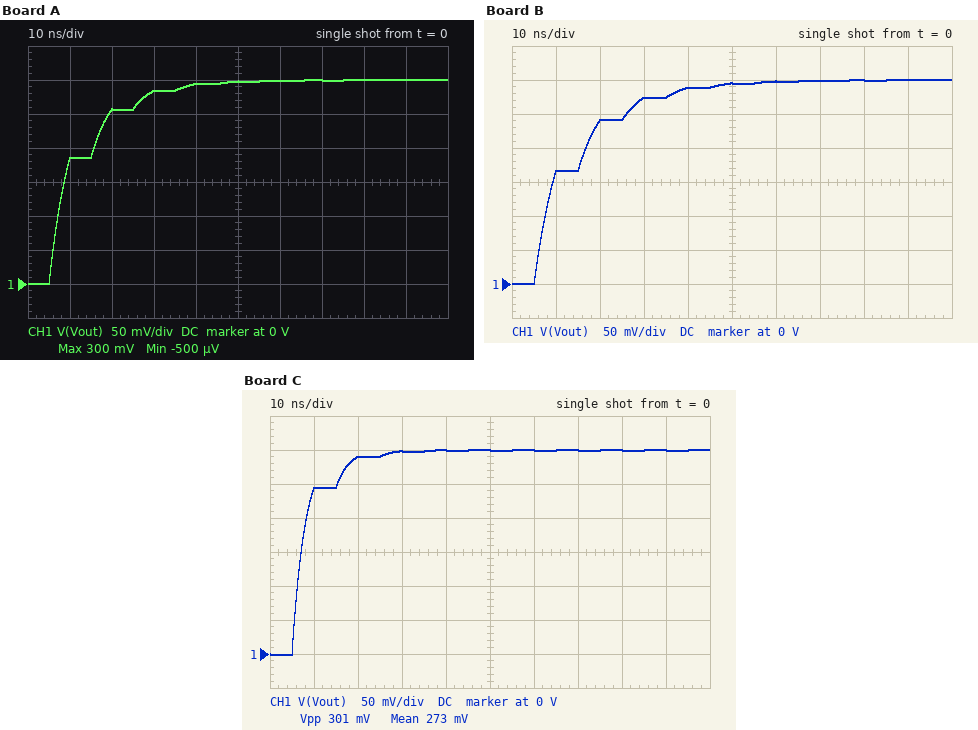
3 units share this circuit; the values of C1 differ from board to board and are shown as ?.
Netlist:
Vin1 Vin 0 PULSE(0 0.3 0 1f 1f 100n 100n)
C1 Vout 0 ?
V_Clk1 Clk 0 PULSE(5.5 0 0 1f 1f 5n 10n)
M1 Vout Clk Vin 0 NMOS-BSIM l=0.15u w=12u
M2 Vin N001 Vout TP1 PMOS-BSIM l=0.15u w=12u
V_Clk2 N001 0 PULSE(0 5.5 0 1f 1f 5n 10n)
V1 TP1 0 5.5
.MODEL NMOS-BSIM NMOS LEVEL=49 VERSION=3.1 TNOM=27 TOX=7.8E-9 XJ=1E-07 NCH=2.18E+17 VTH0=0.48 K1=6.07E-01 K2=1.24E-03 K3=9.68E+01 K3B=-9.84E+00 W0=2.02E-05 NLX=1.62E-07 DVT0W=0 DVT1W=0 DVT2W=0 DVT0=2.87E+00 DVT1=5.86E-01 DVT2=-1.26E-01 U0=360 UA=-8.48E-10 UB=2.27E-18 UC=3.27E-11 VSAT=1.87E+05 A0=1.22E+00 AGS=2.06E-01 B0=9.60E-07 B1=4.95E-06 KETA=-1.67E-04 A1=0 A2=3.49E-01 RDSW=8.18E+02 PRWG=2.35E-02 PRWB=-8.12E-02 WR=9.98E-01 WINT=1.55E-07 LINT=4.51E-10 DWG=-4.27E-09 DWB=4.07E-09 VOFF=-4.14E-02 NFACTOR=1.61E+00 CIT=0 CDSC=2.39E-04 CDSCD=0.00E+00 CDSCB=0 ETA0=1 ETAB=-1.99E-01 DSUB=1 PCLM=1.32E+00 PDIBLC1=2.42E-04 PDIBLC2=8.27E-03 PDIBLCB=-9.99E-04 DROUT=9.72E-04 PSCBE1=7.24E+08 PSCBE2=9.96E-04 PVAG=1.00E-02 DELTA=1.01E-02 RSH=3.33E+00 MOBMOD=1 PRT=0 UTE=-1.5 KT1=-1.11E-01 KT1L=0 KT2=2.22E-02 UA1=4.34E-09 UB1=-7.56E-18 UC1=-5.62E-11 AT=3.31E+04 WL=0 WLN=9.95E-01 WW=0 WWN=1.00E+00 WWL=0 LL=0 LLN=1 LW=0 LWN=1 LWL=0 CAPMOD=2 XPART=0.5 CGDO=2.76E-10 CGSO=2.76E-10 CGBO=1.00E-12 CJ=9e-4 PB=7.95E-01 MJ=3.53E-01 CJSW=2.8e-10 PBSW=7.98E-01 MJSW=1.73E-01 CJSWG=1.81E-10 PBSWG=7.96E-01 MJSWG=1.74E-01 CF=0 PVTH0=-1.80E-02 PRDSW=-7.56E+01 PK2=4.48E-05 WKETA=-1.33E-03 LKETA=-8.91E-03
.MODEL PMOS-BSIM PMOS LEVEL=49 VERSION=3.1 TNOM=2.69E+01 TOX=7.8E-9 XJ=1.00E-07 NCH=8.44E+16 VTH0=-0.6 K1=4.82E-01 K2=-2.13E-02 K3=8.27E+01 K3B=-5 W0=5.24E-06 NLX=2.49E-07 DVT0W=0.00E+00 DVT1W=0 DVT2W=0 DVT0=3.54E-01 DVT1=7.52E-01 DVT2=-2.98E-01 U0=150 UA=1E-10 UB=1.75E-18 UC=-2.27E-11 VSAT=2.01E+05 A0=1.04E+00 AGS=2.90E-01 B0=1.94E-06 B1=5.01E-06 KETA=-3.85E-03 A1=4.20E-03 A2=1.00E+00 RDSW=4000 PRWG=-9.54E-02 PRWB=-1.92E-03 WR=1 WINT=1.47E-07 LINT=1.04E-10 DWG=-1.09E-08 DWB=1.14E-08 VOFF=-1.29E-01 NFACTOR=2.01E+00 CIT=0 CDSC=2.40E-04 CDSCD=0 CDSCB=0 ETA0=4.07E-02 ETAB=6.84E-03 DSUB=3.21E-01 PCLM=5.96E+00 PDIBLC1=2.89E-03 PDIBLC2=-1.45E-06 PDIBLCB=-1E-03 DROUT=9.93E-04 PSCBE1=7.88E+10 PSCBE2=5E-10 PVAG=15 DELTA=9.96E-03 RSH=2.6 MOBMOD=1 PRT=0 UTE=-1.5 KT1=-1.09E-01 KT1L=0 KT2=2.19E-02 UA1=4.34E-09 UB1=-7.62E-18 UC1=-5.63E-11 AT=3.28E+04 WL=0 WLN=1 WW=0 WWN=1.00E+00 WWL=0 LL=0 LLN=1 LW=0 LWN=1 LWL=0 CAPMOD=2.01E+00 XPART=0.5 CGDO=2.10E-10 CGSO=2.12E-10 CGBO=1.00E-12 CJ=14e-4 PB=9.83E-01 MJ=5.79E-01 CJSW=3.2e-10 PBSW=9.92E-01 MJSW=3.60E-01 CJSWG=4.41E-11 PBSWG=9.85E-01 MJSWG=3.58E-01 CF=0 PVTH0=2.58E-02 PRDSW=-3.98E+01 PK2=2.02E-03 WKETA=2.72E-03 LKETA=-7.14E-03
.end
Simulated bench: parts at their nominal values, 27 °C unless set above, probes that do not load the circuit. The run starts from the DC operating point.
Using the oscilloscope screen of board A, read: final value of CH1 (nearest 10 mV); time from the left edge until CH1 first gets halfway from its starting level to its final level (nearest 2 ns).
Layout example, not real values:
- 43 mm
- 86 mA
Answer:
- 300 mV
- 8 ns
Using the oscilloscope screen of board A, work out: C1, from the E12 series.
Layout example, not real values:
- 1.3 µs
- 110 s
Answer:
- 47 pF
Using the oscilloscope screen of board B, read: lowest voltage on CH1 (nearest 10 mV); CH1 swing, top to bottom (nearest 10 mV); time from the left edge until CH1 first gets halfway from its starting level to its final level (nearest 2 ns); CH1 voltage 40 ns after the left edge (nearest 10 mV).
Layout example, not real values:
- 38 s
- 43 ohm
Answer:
- 0 V
- 300 mV
- 10 ns
- 290 mV
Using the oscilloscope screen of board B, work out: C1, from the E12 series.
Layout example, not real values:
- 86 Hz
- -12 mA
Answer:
- 56 pF
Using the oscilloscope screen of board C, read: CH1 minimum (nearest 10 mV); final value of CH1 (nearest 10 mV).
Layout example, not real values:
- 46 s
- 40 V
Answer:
- 0 V
- 300 mV
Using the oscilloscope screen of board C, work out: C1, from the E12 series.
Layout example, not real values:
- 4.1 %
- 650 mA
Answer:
- 27 pF
